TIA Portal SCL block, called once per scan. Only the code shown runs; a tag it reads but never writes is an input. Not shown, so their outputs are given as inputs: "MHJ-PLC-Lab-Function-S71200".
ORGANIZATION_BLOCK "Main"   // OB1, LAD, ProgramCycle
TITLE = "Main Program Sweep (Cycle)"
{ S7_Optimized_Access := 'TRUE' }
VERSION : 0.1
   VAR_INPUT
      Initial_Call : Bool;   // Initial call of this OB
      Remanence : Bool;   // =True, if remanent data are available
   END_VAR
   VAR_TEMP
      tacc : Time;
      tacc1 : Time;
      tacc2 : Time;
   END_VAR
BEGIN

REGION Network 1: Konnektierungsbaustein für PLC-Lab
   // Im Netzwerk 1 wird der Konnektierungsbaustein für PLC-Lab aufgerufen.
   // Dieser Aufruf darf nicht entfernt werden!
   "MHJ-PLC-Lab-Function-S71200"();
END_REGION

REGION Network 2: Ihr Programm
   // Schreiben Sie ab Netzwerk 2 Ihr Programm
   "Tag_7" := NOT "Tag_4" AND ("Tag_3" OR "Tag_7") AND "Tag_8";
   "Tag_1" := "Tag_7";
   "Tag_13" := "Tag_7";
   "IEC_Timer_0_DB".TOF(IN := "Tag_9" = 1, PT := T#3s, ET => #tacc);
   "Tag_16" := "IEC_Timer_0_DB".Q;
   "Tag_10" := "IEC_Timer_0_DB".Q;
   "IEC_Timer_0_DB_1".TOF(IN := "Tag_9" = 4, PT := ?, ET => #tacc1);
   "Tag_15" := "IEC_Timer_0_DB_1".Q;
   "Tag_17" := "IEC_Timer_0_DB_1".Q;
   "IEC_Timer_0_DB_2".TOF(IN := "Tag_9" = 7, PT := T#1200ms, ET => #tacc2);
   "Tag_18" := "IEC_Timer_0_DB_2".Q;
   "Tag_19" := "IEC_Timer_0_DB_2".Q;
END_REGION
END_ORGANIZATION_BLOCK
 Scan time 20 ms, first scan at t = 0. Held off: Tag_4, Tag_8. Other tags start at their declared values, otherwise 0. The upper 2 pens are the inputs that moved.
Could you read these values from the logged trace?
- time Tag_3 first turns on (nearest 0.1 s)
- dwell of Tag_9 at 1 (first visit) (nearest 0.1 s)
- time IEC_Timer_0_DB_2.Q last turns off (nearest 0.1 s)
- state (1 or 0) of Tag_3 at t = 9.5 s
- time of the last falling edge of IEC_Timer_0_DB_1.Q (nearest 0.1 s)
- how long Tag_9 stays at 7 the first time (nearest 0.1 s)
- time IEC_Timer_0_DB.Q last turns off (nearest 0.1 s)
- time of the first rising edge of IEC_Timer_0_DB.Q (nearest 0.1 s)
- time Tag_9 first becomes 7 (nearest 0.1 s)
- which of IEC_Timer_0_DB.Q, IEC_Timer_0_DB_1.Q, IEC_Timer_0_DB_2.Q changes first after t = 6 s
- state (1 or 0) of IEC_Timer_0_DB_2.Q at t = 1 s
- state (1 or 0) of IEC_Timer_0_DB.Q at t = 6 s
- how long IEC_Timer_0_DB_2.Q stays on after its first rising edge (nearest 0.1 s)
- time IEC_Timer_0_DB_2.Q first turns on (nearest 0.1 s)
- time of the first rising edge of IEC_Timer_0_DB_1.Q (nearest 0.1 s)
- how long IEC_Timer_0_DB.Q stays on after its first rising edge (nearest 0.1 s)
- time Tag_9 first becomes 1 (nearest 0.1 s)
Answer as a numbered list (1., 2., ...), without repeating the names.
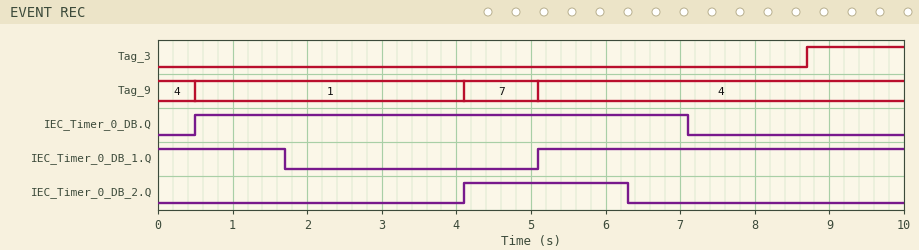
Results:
1. 8.7 s
2. 3.6 s
3. 6.3 s
4. 1
5. 1.7 s
6. 1.0 s
7. 7.1 s
8. 0.5 s
9. 4.1 s
10. IEC_Timer_0_DB_2.Q
11. 0
12. 1
13. 2.2 s
14. 4.1 s
15. 5.1 s
16. 6.6 s
17. 0.5 s
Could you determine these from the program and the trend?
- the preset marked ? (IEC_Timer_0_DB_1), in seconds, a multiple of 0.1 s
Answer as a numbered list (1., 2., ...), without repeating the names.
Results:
1. 1.2 s
